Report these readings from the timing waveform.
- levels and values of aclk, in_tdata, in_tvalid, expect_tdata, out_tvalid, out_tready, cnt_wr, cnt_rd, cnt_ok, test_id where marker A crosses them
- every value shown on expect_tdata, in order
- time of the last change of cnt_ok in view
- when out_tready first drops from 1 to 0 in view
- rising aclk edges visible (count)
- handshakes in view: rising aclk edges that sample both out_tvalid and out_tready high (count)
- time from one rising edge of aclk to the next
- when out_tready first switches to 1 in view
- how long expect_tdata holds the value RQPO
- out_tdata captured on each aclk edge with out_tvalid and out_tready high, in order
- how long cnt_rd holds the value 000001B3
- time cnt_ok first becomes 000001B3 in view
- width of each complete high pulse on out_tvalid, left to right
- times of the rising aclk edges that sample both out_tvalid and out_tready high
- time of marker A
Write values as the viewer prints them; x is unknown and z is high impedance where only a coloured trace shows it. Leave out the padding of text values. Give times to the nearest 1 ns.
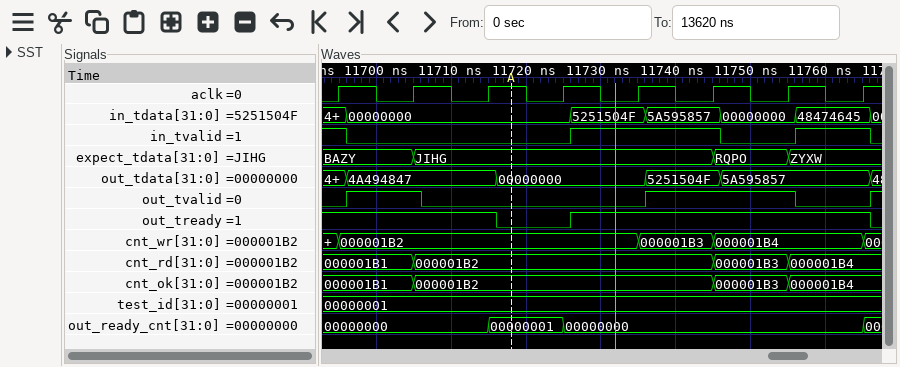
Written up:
aclk=1, in_tdata=00000000, in_tvalid=0, expect_tdata=JIHG, out_tvalid=0, out_tready=0, cnt_wr=000001B2, cnt_rd=000001B2, cnt_ok=000001B2, test_id=00000001
BAZY, JIHG, RQPO, ZYXW
11755 ns
11716 ns
8
3
10 ns
11726 ns
10 ns
4A494847, 5251504F, 5A595857
10 ns
11745 ns
10 ns, 20 ns
11705 ns, 11745 ns, 11755 ns
11718 ns
